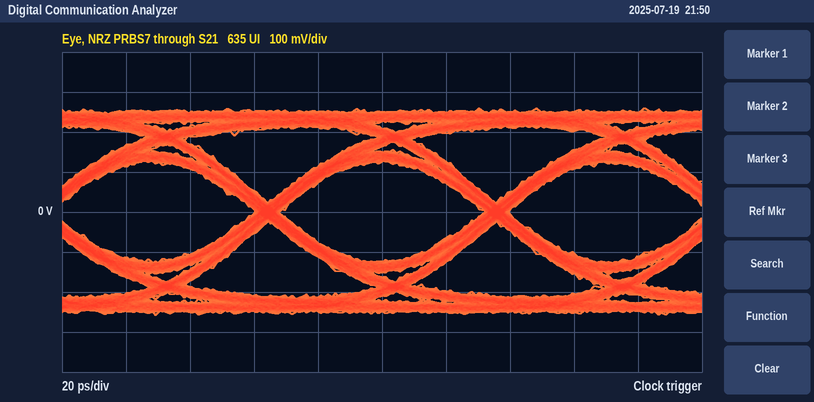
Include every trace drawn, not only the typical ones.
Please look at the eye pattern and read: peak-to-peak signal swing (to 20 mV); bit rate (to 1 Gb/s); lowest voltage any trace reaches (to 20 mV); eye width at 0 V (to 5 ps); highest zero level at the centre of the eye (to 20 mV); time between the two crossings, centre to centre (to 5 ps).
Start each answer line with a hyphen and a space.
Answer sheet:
- 520 mV
- 14 Gb/s
- -260 mV
- 65 ps
- -120 mV
- 70 ps
